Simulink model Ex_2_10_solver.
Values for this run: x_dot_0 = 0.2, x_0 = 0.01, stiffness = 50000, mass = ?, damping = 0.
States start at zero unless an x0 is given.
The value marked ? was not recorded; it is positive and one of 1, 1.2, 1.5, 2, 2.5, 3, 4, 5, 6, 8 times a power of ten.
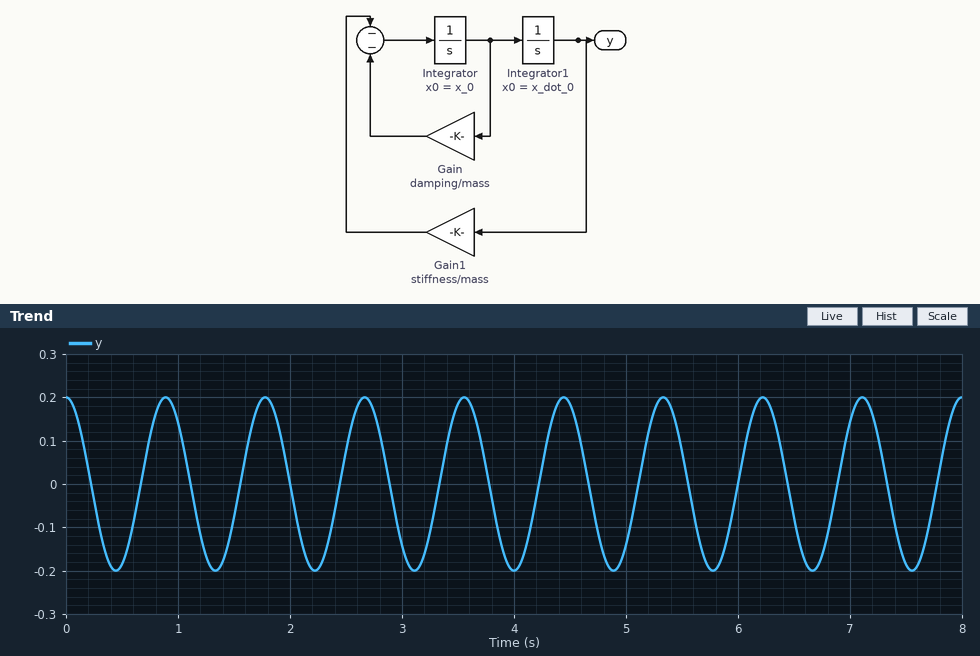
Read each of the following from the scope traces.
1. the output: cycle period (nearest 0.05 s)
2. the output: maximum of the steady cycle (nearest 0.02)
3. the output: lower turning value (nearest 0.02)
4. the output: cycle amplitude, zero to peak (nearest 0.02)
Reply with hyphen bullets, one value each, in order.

- 0.90 s
- 0.20
- -0.20
- 0.20
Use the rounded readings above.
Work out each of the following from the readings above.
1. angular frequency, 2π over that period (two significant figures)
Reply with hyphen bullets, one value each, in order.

- 7.0 rad/s
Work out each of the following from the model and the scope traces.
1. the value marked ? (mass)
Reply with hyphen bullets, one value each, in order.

- 1000
